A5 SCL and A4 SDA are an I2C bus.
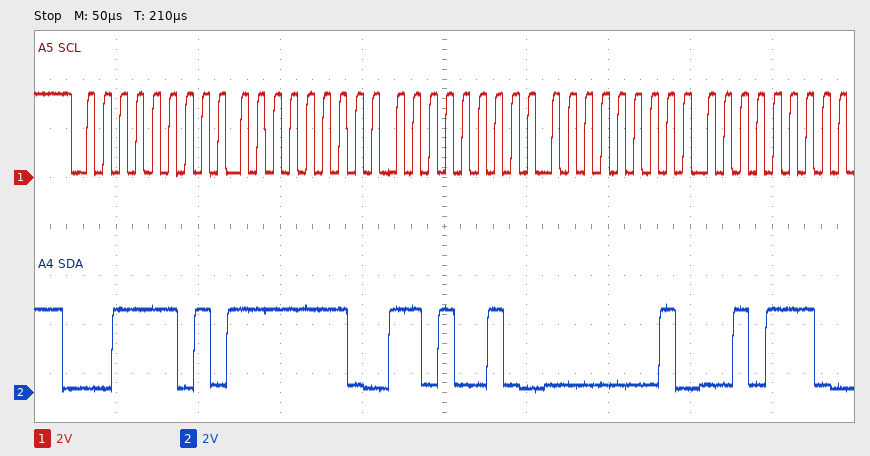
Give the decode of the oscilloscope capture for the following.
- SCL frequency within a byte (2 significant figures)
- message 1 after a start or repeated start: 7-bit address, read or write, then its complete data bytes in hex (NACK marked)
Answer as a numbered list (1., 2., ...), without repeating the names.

1. 100 kHz
2. 0x1E read: FE D2 01 2E
